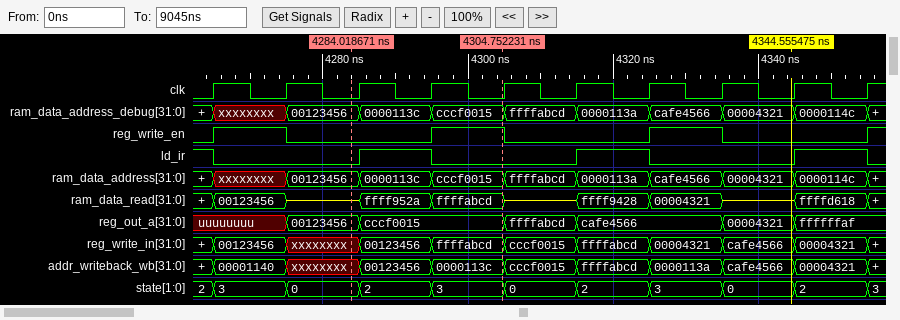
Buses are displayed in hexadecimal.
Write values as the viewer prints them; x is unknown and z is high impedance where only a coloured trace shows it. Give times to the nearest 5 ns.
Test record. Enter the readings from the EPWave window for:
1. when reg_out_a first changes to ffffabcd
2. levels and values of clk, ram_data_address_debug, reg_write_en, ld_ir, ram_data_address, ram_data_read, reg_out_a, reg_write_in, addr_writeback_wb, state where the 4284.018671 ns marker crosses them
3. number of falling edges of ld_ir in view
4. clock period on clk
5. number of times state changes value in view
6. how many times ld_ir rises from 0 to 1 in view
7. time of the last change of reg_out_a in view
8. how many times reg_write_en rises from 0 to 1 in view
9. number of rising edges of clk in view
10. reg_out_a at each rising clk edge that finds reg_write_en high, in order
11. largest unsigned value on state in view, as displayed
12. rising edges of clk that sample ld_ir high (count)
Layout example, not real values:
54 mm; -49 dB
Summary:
4305 ns; clk=0, ram_data_address_debug=00123456, reg_write_en=0, ld_ir=0, ram_data_address=00123456, ram_data_read=z, reg_out_a=00123456, reg_write_in=xxxxxxxx, addr_writeback_wb=xxxxxxxx, state=0; 4; 10 ns; 10; 3; 4345 ns; 4; 10; uuuuuuuu, cccf0015, cafe4566; 3; 4
